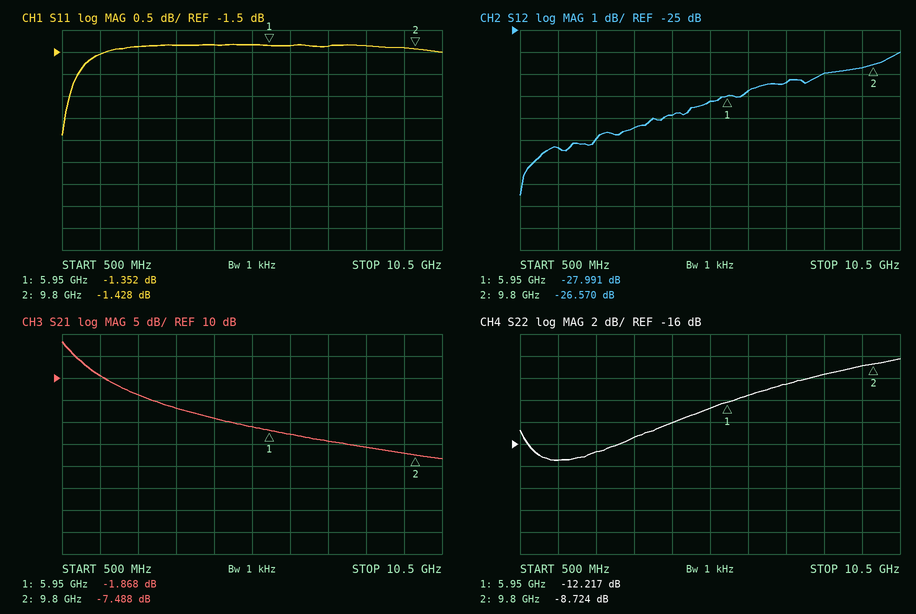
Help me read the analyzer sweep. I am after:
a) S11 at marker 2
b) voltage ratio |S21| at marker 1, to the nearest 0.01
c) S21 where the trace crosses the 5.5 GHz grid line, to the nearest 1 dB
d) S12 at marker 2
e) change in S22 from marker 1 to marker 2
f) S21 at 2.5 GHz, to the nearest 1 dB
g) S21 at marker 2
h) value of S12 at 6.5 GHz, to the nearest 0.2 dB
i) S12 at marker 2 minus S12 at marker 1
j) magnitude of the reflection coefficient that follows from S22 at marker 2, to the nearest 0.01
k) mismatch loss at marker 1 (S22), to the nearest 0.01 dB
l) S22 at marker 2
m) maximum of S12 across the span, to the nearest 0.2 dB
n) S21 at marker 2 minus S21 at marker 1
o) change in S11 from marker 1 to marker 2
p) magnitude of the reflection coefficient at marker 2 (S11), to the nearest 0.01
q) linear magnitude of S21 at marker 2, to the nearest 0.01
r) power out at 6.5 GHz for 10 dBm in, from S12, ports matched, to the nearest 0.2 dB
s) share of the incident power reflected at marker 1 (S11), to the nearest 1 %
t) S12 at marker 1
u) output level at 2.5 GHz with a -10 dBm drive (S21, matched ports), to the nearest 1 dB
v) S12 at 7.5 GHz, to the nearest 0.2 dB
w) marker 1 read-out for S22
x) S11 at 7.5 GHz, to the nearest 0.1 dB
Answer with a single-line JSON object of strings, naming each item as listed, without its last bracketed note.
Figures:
{"S11 at marker 2": "-1.428 dB", "voltage ratio |S21| at marker 1, to the nearest 0.01": "0.81", "S21 where the trace crosses the 5.5 GHz grid line, to the nearest 1 dB": "-1 dB", "S12 at marker 2": "-26.570 dB", "change in S22 from marker 1 to marker 2": "3.493 dB", "S21 at 2.5 GHz, to the nearest 1 dB": "6 dB", "S21 at marker 2": "-7.488 dB", "value of S12 at 6.5 GHz, to the nearest 0.2 dB": "-27.8 dB", "S12 at marker 2 minus S12 at marker 1": "1.421 dB", "magnitude of the reflection coefficient that follows from S22 at marker 2, to the nearest 0.01": "0.37", "mismatch loss at marker 1 (S22), to the nearest 0.01 dB": "0.27 dB", "S22 at marker 2": "-8.724 dB", "maximum of S12 across the span, to the nearest 0.2 dB": "-26.0 dB", "S21 at marker 2 minus S21 at marker 1": "-5.620 dB", "change in S11 from marker 1 to marker 2": "-0.076 dB", "magnitude of the reflection coefficient at marker 2 (S11), to the nearest 0.01": "0.85", "linear magnitude of S21 at marker 2, to the nearest 0.01": "0.42", "power out at 6.5 GHz for 10 dBm in, from S12, ports matched, to the nearest 0.2 dB": "-17.8 dBm", "share of the incident power reflected at marker 1 (S11), to the nearest 1 %": "73 %", "S12 at marker 1": "-27.991 dB", "output level at 2.5 GHz with a -10 dBm drive (S21, matched ports), to the nearest 1 dB": "-4 dBm", "S12 at 7.5 GHz, to the nearest 0.2 dB": "-27.4 dB", "marker 1 read-out for S22": "-12.217 dB", "S11 at 7.5 GHz, to the nearest 0.1 dB": "-1.4 dB"}
